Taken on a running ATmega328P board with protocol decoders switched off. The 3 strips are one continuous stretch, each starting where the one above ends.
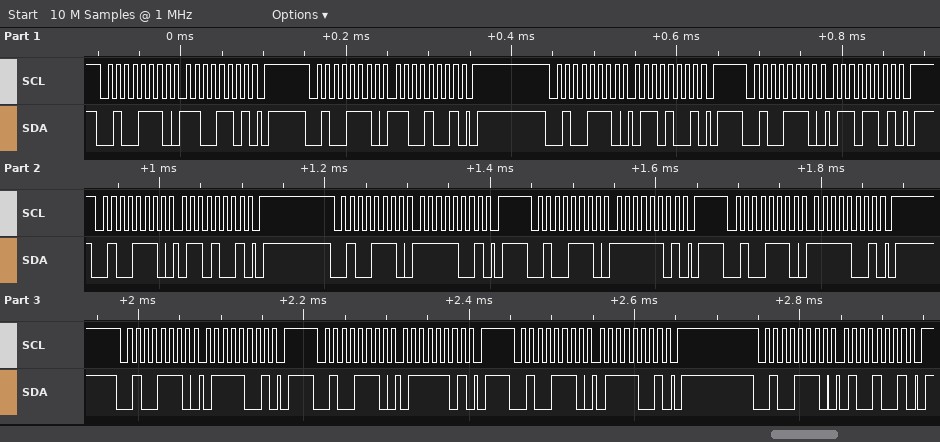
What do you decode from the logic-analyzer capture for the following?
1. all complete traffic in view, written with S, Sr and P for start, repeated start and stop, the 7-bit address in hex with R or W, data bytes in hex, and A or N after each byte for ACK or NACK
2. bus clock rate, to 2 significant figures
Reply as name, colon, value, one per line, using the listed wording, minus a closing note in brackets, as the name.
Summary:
all complete traffic in view, written with S, Sr and P for start, repeated start and stop, the 7-bit address in hex with R or W, data bytes in hex, and A or N after each byte for ACK or NACK: S 27W A CD A P S 27W A C9 A P S 27W A 69 A P S 27W A 6D A P S 27W A 69 A P S 27W A F9 A P S 27W A FD A P S 27W A F9 A P S 27W A 79 A P S 27W A 7D A P S 27W A 79 A P S 27W A 49 A P
bus clock rate, to 2 significant figures: 100 kHz
